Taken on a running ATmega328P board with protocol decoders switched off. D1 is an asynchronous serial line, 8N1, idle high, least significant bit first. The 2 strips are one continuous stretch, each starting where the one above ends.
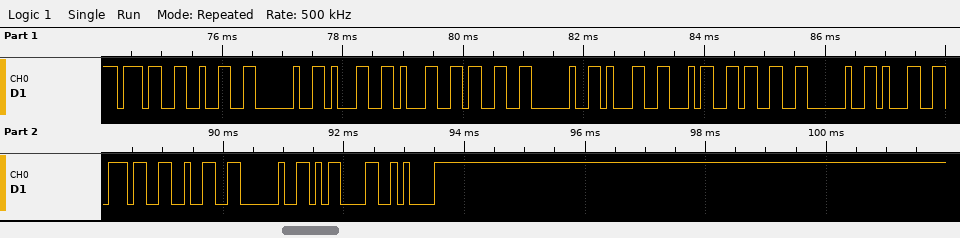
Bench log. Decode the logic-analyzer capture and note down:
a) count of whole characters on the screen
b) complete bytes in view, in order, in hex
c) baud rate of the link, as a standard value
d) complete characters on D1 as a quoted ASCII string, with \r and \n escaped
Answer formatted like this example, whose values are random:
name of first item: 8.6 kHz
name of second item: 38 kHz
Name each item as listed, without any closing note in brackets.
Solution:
count of whole characters on the screen: 17
complete bytes in view, in order, in hex: 37 32 20 31 31 33 20 31 34 33 20 31 37 32 20 0D 0A
baud rate of the link, as a standard value: 9600 baud
complete characters on D1 as a quoted ASCII string, with \r and \n escaped: "72 113 143 172 \r\n"
